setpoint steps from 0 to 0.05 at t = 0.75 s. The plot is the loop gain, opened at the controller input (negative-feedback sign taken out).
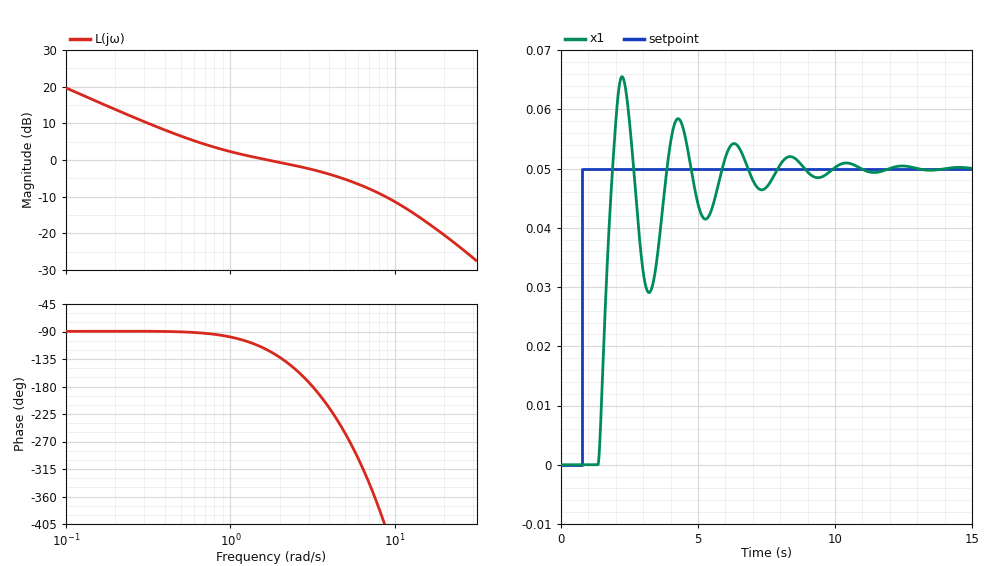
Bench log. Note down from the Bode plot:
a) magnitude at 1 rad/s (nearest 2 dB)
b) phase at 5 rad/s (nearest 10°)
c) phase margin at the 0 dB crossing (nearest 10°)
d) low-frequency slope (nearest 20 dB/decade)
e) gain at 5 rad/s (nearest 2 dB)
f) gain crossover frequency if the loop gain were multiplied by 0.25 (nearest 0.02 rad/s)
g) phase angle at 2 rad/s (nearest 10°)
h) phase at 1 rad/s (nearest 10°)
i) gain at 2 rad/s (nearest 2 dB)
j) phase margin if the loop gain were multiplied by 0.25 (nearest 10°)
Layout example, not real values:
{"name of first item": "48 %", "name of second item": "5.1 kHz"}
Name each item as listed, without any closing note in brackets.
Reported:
{"magnitude at 1 rad/s": "2 dB", "phase at 5 rad/s": "-260°", "phase margin at the 0 dB crossing": "60°", "low-frequency slope": "-20 dB/decade", "gain at 5 rad/s": "-6 dB", "gain crossover frequency if the loop gain were multiplied by 0.25": "0.24 rad/s", "phase angle at 2 rad/s": "-130°", "phase at 1 rad/s": "-100°", "gain at 2 rad/s": "0 dB", "phase margin if the loop gain were multiplied by 0.25": "90°"}
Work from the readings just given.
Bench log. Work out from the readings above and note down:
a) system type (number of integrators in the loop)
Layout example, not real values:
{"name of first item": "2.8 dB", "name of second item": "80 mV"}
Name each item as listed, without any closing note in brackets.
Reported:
{"system type": "1"}
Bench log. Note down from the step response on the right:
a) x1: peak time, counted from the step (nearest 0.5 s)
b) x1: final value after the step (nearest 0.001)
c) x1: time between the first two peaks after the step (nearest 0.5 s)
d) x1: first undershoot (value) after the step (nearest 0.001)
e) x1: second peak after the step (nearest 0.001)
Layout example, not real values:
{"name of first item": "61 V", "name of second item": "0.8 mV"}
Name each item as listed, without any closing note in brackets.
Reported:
{"x1: peak time, counted from the step": "1.5 s", "x1: final value after the step": "0.050", "x1: time between the first two peaks after the step": "2.0 s", "x1: first undershoot (value) after the step": "0.029", "x1: second peak after the step": "0.058"}
